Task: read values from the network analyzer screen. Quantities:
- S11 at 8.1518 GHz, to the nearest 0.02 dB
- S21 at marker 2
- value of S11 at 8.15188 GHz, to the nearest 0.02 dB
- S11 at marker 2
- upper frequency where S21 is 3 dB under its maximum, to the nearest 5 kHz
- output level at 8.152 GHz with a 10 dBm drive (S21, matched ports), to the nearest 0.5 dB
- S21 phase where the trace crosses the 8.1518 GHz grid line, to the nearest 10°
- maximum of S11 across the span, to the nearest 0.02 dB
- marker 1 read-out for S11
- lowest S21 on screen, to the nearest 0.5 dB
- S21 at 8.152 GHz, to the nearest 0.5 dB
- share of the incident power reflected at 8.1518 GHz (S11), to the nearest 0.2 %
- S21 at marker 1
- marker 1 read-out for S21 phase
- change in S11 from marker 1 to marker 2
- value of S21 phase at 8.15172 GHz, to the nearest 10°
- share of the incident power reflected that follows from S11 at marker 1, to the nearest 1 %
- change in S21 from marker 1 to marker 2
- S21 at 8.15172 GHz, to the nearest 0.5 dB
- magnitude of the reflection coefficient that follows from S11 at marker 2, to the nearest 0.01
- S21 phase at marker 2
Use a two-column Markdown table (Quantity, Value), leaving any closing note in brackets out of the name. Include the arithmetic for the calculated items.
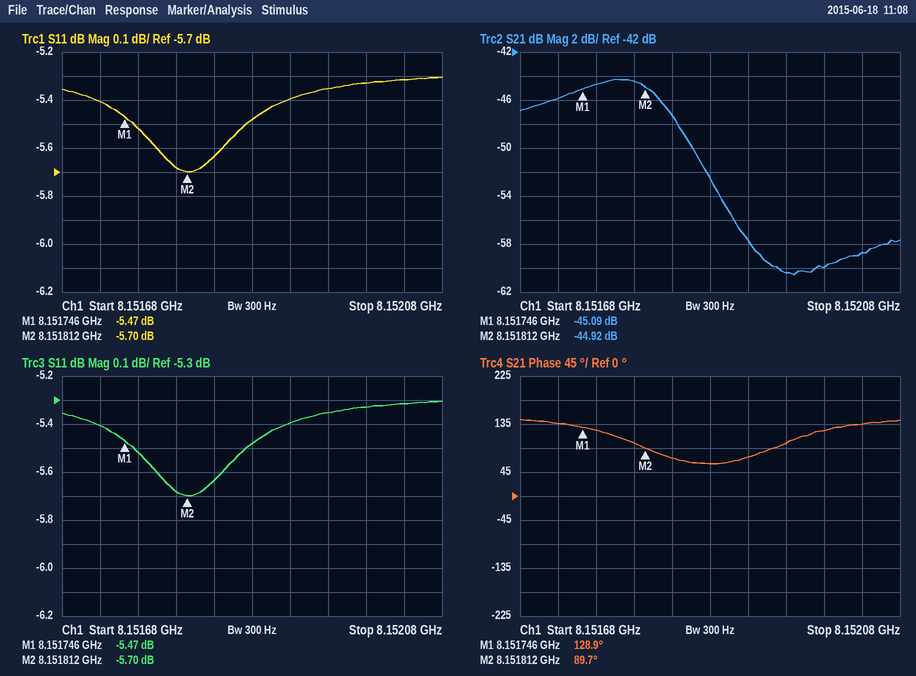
| Quantity | Value |
|---|---|
| S11 at 8.1518 GHz, to the nearest 0.02 dB | -5.68 dB |
| S21 at marker 2 | -44.92 dB |
| value of S11 at 8.15188 GHz, to the nearest 0.02 dB | -5.48 dB |
| S11 at marker 2 | -5.70 dB |
| upper frequency where S21 is 3 dB under its maximum, to the nearest 5 kHz | 8.151840 GHz |
| output level at 8.152 GHz with a 10 dBm drive (S21, matched ports), to the nearest 0.5 dB | 10 dBm + (-60.0 dB) = -50.0 dBm |
| S21 phase where the trace crosses the 8.1518 GHz grid line, to the nearest 10° | 100° |
| maximum of S11 across the span, to the nearest 0.02 dB | -5.30 dB |
| marker 1 read-out for S11 | -5.47 dB |
| lowest S21 on screen, to the nearest 0.5 dB | -60.5 dB |
| S21 at 8.152 GHz, to the nearest 0.5 dB | -60.0 dB |
| share of the incident power reflected at 8.1518 GHz (S11), to the nearest 0.2 % | 10^(-5.68/10) ≈ 27.0 % |
| S21 at marker 1 | -45.09 dB |
| marker 1 read-out for S21 phase | 128.9° |
| change in S11 from marker 1 to marker 2 | -5.7 − (-5.47) = -0.23 dB |
| value of S21 phase at 8.15172 GHz, to the nearest 10° | 140° |
| share of the incident power reflected that follows from S11 at marker 1, to the nearest 1 % | 10^(-5.47/10) ≈ 28 % |
| change in S21 from marker 1 to marker 2 | -44.92 − (-45.09) = 0.17 dB |
| S21 at 8.15172 GHz, to the nearest 0.5 dB | -46.0 dB |
| magnitude of the reflection coefficient that follows from S11 at marker 2, to the nearest 0.01 | 10^(-5.7/20) ≈ 0.52 |
| S21 phase at marker 2 | 89.7° |
